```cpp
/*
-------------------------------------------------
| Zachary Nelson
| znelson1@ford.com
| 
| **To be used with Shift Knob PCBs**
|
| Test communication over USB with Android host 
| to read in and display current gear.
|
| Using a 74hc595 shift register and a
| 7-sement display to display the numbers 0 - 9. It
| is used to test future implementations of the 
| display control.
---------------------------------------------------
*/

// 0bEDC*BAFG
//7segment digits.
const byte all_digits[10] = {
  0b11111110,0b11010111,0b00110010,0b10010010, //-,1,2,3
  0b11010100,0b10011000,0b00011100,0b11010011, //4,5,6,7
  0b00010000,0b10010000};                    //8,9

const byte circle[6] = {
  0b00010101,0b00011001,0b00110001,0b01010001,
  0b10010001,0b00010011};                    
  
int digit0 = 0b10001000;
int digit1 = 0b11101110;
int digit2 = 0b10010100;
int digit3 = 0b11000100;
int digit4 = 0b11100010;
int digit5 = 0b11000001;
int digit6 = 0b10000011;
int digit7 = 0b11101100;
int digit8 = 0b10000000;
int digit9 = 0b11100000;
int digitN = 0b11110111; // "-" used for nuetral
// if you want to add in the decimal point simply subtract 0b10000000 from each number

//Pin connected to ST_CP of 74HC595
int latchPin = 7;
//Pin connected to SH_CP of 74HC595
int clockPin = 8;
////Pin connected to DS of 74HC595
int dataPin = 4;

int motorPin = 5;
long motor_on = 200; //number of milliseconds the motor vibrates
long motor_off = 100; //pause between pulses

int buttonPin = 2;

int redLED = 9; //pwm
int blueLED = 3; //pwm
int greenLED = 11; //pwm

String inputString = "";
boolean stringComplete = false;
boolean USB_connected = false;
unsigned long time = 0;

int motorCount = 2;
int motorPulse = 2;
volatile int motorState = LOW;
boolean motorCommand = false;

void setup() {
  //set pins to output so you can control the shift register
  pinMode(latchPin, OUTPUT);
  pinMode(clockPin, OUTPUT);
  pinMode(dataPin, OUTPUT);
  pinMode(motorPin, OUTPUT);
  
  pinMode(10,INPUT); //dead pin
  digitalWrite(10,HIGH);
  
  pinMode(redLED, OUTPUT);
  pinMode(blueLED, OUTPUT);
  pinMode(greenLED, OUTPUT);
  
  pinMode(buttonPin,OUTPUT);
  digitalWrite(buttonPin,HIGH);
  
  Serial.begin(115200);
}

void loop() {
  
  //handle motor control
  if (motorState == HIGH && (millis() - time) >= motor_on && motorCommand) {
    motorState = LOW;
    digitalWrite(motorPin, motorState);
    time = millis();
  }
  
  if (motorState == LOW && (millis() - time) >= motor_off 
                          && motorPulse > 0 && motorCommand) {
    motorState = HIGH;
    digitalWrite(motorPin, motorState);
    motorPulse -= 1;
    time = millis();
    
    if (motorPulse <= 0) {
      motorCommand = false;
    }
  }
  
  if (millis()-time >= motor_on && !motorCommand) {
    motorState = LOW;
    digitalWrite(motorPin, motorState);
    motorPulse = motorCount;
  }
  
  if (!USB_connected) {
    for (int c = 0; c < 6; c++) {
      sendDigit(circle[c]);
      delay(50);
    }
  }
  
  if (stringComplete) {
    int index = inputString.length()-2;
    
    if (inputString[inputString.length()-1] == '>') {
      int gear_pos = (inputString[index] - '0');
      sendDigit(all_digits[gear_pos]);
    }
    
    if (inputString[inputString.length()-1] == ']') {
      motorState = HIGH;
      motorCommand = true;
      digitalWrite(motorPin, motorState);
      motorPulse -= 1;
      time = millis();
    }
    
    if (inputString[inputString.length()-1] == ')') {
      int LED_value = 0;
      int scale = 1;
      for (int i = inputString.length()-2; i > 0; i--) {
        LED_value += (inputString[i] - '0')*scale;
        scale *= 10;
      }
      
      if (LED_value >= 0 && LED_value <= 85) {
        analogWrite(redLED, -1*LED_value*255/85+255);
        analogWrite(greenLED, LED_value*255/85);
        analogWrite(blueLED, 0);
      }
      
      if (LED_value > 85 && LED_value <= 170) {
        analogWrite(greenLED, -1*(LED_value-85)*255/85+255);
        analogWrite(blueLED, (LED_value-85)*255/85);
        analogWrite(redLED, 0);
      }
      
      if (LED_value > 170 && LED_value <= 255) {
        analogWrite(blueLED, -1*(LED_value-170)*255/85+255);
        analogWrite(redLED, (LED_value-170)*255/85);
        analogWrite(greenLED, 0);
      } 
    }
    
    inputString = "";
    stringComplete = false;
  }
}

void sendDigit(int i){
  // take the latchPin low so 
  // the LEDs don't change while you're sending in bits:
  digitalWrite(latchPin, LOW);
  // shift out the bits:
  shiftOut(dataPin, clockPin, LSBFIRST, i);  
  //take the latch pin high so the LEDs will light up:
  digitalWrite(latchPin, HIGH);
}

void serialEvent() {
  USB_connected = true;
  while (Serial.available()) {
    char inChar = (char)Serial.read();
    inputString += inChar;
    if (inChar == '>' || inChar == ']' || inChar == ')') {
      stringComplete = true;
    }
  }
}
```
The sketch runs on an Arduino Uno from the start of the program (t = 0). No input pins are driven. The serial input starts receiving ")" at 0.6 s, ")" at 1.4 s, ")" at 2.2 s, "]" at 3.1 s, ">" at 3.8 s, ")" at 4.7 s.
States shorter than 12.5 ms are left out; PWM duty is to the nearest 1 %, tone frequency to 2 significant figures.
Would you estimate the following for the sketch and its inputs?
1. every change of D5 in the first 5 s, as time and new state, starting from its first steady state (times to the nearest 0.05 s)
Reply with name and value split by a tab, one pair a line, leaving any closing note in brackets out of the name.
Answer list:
every change of D5 in the first 5 s, as time and new state, starting from its first steady state	0 s low; 3.1 s high; 3.3 s low; 3.4 s high; 3.6 s low
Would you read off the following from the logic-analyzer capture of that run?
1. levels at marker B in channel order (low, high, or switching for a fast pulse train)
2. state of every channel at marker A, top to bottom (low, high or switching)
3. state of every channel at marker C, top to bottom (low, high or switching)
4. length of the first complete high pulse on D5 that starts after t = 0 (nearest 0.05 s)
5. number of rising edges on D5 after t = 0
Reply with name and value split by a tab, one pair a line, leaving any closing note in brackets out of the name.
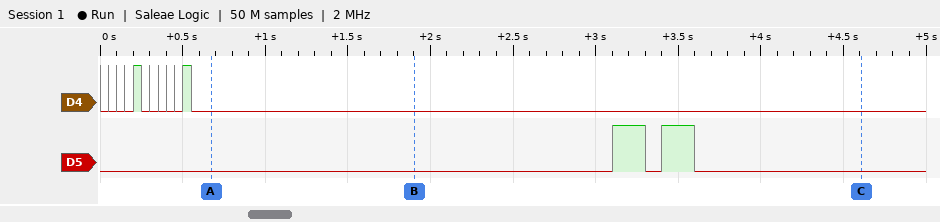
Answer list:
levels at marker B in channel order	D4 low, D5 low
state of every channel at marker A, top to bottom	D4 low, D5 low
state of every channel at marker C, top to bottom	D4 low, D5 low
length of the first complete high pulse on D5 that starts after t = 0	0.20 s
number of rising edges on D5 after t = 0	2
